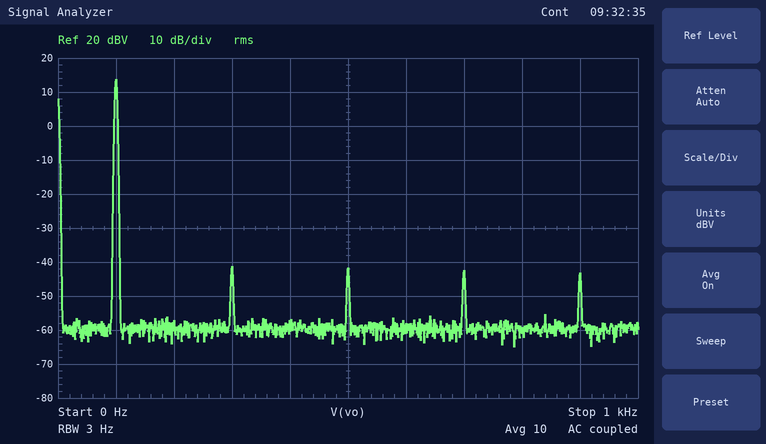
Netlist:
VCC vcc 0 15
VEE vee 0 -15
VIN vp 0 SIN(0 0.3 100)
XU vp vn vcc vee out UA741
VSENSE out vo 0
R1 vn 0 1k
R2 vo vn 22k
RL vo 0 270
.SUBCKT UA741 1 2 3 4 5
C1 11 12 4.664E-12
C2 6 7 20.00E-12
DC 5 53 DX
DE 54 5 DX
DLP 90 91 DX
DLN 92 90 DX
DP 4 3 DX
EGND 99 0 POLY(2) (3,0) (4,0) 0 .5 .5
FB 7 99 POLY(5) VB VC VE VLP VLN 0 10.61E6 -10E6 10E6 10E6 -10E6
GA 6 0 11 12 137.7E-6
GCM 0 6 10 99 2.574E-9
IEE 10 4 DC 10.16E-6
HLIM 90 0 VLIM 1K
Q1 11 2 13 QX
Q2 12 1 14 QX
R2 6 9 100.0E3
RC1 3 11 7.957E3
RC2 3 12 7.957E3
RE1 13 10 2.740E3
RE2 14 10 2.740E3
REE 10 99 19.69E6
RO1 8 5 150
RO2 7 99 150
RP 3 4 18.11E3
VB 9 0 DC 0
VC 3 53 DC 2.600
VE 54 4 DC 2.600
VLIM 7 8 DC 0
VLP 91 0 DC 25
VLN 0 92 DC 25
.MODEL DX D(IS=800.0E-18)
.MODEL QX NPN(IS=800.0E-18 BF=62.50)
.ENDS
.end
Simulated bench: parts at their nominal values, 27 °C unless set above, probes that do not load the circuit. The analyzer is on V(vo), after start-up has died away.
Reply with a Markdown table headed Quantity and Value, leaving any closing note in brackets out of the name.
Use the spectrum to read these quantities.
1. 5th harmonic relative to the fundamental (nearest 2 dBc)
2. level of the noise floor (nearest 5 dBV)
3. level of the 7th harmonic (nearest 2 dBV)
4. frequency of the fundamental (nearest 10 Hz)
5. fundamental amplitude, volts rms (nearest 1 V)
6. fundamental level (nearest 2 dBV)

| Quantity | Value |
|---|---|
| 5th harmonic relative to the fundamental | -56 dBc |
| level of the noise floor | -60 dBV |
| level of the 7th harmonic | -42 dBV |
| frequency of the fundamental | 100 Hz |
| fundamental amplitude, volts rms | 5 V |
| fundamental level | 14 dBV |
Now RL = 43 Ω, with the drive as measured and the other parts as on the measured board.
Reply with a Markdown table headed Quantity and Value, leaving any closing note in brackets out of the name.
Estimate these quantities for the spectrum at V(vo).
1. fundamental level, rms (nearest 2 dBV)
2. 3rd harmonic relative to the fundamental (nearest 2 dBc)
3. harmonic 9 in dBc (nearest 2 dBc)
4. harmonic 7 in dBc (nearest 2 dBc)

| Quantity | Value |
|---|---|
| fundamental level, rms | 0 dBV |
| 3rd harmonic relative to the fundamental | -10 dBc |
| harmonic 9 in dBc | -22 dBc |
| harmonic 7 in dBc | -18 dBc |
